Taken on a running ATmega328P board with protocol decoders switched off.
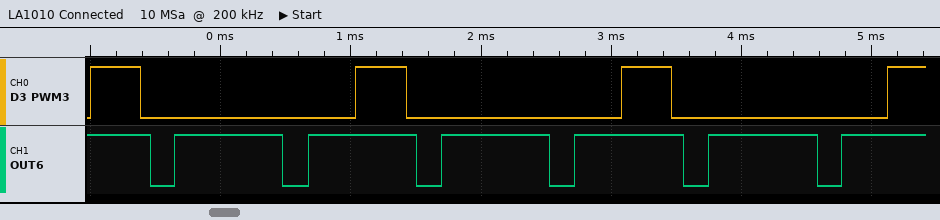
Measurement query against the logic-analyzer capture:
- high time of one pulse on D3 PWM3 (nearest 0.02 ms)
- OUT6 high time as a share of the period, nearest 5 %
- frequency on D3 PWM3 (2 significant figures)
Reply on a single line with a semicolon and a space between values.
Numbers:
0.38 ms; 80 %; 490 Hz
